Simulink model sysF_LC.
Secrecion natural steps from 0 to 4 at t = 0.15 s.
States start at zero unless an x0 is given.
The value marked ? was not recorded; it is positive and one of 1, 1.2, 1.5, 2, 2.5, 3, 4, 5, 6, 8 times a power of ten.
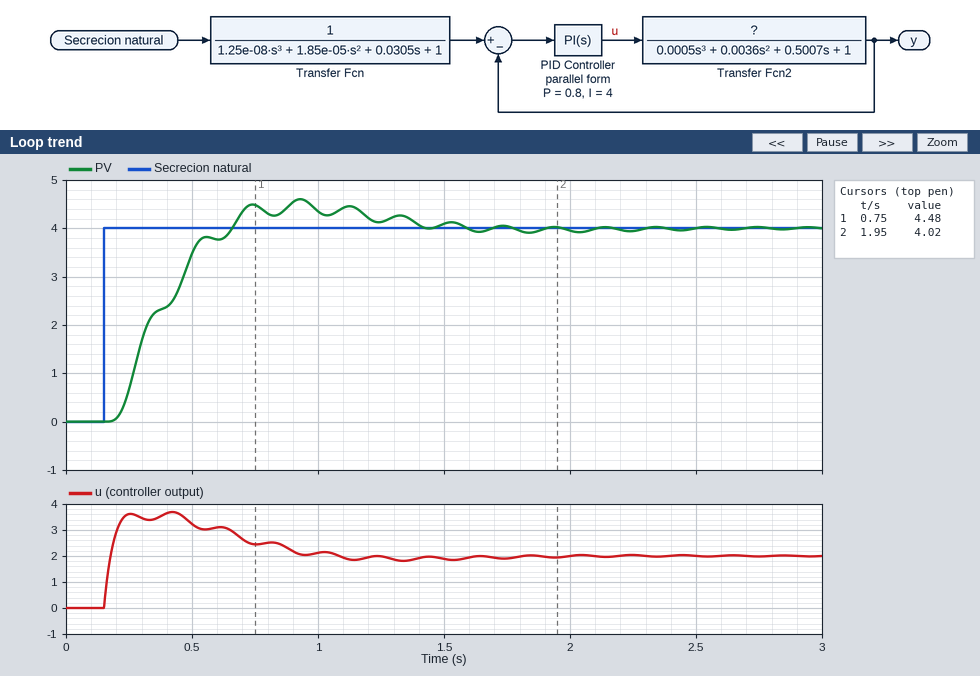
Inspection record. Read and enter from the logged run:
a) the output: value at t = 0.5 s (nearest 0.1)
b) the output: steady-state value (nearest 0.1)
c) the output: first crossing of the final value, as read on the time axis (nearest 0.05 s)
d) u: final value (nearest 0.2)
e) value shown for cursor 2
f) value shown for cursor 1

3.5
4.0
0.65 s
2.0
4.02
4.48
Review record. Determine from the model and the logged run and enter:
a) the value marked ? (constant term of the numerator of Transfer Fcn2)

2
